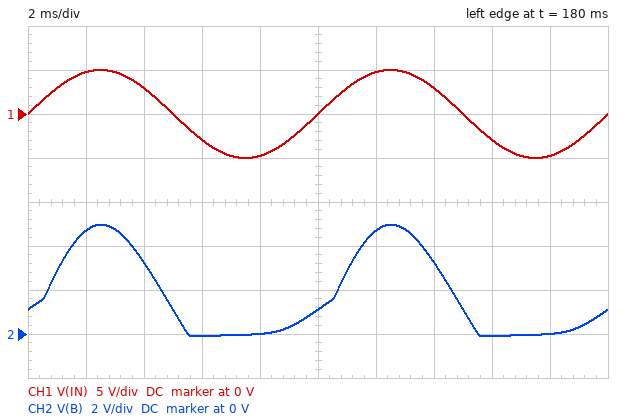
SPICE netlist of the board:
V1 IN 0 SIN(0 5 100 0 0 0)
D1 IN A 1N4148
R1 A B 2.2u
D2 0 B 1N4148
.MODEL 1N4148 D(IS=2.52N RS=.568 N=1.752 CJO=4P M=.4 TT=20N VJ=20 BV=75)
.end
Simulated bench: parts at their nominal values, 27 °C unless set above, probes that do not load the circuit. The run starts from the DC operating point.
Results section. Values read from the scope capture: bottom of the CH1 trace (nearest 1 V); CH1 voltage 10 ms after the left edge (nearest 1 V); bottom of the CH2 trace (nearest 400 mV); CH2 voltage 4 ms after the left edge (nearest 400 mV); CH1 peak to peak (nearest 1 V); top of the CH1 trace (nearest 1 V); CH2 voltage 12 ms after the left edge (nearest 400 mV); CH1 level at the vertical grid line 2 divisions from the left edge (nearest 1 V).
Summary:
-5 V
0 V
0 V
3.2 V
10 V
5 V
4.8 V
3 V
